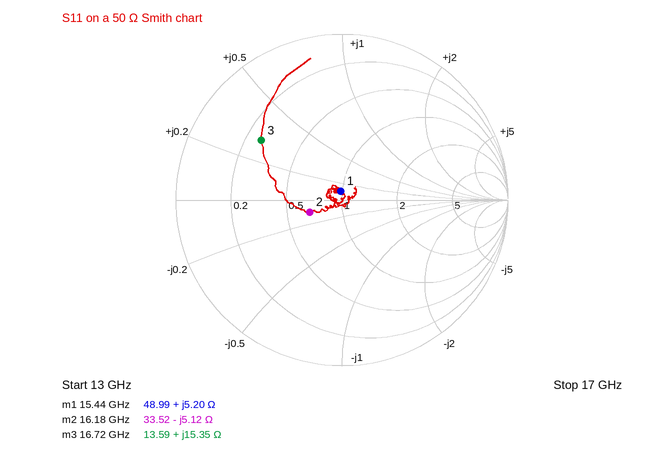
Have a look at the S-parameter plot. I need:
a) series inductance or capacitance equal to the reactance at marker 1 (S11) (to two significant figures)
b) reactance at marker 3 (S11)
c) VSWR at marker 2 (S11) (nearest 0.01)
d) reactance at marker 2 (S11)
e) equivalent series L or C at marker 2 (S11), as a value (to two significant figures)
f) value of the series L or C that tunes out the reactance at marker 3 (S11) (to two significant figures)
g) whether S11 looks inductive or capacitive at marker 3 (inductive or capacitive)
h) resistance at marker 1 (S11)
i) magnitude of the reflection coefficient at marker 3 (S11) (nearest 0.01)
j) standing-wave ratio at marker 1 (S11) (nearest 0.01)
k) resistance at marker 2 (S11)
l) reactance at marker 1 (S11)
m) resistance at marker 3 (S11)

54 pH
+15.35 Ω
1.52
-5.12 Ω
1.9 pF
620 fF
inductive
48.99 Ω
0.60
1.11
33.52 Ω
+5.20 Ω
13.59 Ω
